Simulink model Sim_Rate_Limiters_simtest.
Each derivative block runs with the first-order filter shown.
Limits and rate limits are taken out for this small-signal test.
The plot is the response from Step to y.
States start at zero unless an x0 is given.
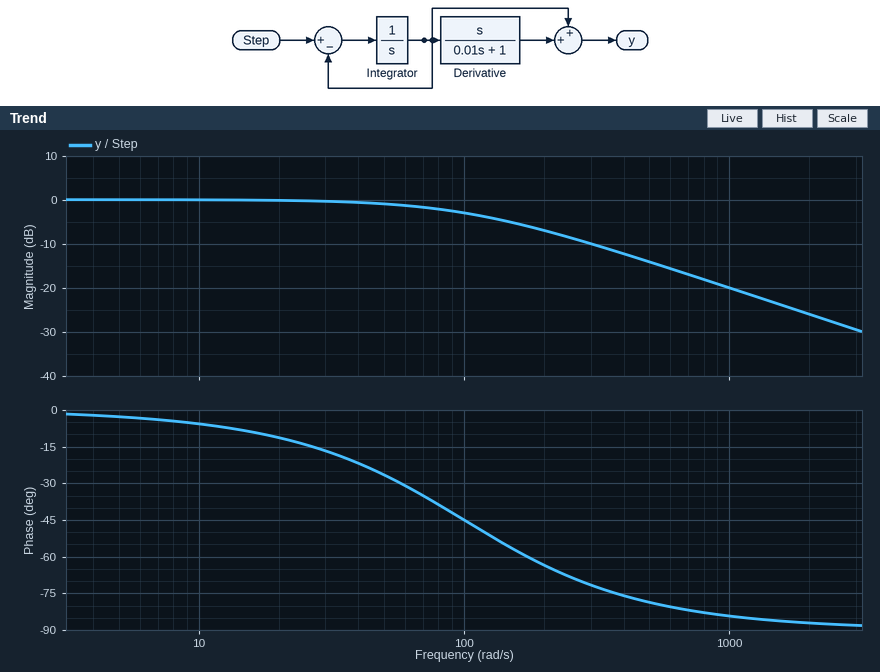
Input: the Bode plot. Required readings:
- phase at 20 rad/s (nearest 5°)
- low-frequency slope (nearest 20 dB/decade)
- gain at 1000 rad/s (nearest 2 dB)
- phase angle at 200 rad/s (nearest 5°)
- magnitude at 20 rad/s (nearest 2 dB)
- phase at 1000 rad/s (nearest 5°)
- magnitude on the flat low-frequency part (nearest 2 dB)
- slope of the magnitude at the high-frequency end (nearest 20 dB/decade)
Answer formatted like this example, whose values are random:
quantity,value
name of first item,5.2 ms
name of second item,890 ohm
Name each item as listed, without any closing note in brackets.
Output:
quantity,value
phase at 20 rad/s,-10°
low-frequency slope,0 dB/decade
gain at 1000 rad/s,-20 dB
phase angle at 200 rad/s,-65°
magnitude at 20 rad/s,0 dB
phase at 1000 rad/s,-85°
magnitude on the flat low-frequency part,0 dB
slope of the magnitude at the high-frequency end,-20 dB/decade
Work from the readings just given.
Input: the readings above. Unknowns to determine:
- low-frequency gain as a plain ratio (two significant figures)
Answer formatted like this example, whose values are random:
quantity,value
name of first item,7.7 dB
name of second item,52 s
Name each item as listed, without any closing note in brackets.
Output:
quantity,value
low-frequency gain as a plain ratio,1.0
